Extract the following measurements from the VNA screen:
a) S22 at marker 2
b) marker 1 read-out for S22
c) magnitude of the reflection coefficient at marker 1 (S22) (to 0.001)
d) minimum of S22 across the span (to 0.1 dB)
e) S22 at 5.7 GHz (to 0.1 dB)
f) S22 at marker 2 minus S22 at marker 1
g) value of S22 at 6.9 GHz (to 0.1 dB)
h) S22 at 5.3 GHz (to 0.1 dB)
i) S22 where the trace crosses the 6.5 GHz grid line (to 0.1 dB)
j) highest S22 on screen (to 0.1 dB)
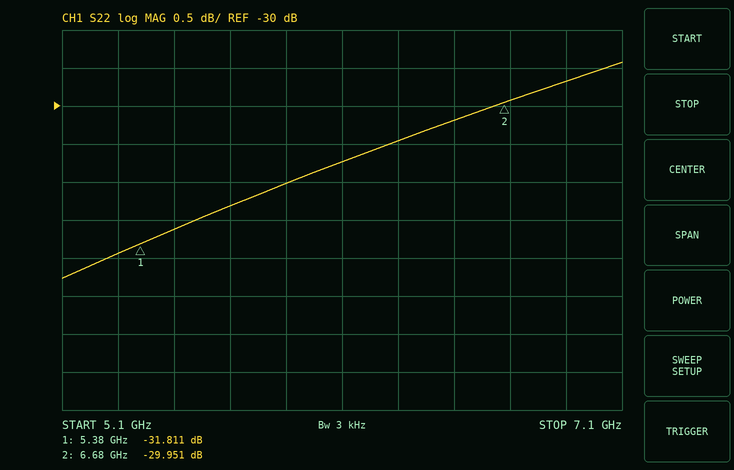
-29.951 dB
-31.811 dB
0.026
-32.3 dB
-31.3 dB
1.860 dB
-29.7 dB
-31.9 dB
-30.2 dB
-29.4 dB
